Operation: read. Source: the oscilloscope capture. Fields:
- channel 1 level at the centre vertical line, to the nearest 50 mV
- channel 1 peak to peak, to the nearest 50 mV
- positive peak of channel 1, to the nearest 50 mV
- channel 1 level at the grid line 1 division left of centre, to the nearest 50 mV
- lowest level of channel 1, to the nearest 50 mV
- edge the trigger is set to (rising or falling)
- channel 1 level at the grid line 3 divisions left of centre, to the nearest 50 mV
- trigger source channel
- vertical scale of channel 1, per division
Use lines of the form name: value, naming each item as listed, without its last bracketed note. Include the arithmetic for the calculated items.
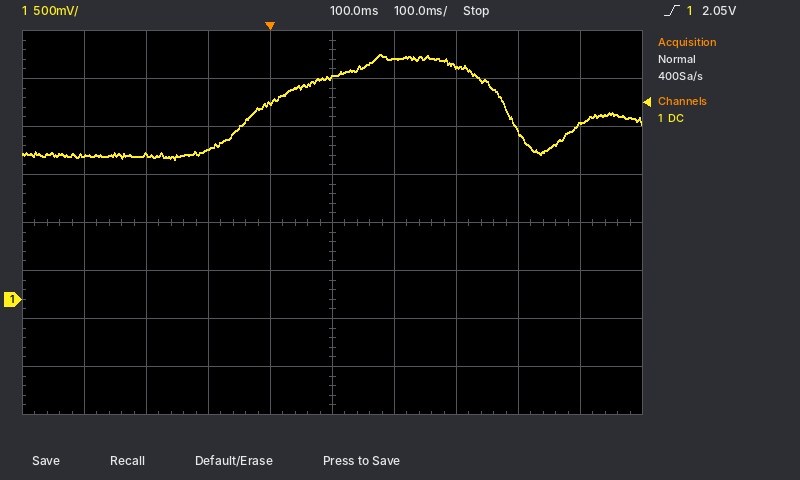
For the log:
channel 1 level at the centre vertical line, to the nearest 50 mV: 2.30 V
channel 1 peak to peak, to the nearest 50 mV: 2.55 V − (1.45 V) = 1.10 V
positive peak of channel 1, to the nearest 50 mV: 2.55 V
channel 1 level at the grid line 1 division left of centre, to the nearest 50 mV: 2.05 V
lowest level of channel 1, to the nearest 50 mV: 1.45 V
edge the trigger is set to: rising
channel 1 level at the grid line 3 divisions left of centre, to the nearest 50 mV: 1.50 V
trigger source channel: channel 1
vertical scale of channel 1, per division: 500 mV
